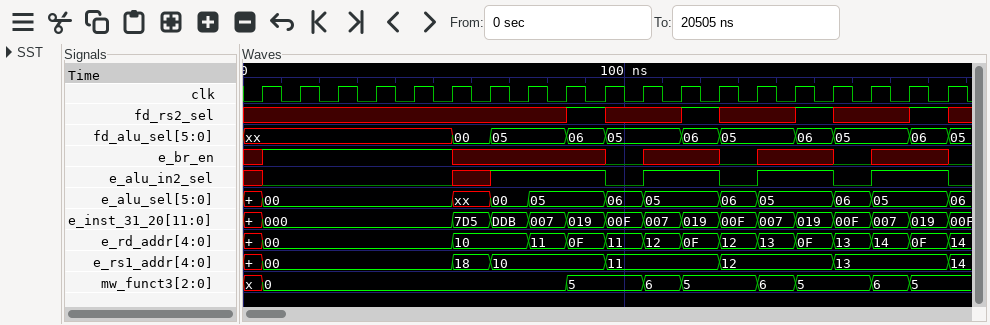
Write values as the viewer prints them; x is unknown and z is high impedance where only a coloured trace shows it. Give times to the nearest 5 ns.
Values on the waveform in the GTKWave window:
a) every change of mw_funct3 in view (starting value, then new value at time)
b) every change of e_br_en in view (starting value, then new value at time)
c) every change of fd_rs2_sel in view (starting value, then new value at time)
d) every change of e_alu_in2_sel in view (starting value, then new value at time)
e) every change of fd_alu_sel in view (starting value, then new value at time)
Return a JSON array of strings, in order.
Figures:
["x, 0 at 5 ns, 5 at 85 ns, 6 at 105 ns, 5 at 115 ns, 6 at 135 ns, 5 at 145 ns, 6 at 165 ns, 5 at 175 ns", "x, 1 at 5 ns, x at 55 ns, 0 at 95 ns, x at 105 ns, 0 at 125 ns, x at 135 ns, 0 at 155 ns, x at 165 ns, 0 at 185 ns", "x, 1 at 85 ns, x at 95 ns, 1 at 115 ns, x at 125 ns, 1 at 145 ns, x at 155 ns, 1 at 175 ns, x at 185 ns", "x, 0 at 5 ns, x at 55 ns, 1 at 65 ns, 0 at 95 ns, 1 at 105 ns, 0 at 125 ns, 1 at 135 ns, 0 at 155 ns, 1 at 165 ns, 0 at 185 ns", "xx, 00 at 55 ns, 05 at 65 ns, 06 at 85 ns, 05 at 95 ns, 06 at 115 ns, 05 at 125 ns, 06 at 145 ns, 05 at 155 ns, 06 at 175 ns, 05 at 185 ns"]
